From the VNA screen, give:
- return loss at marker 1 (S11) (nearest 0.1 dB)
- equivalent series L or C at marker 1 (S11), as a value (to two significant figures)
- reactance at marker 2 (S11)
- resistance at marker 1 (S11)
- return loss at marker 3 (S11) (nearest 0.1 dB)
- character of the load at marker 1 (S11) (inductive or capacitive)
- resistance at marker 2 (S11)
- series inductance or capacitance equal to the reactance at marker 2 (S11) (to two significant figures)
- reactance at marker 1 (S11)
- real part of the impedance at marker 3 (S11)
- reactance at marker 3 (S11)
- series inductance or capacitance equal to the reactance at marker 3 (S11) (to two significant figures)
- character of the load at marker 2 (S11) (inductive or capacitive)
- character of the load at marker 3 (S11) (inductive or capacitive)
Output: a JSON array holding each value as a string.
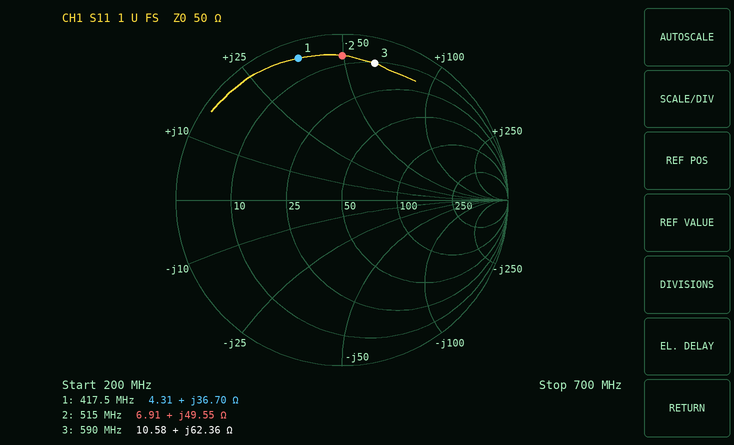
["1.0 dB", "14 nH", "+49.55 Ω", "4.31 Ω", "1.4 dB", "inductive", "6.91 Ω", "15 nH", "+36.70 Ω", "10.58 Ω", "+62.36 Ω", "17 nH", "inductive", "inductive"]
